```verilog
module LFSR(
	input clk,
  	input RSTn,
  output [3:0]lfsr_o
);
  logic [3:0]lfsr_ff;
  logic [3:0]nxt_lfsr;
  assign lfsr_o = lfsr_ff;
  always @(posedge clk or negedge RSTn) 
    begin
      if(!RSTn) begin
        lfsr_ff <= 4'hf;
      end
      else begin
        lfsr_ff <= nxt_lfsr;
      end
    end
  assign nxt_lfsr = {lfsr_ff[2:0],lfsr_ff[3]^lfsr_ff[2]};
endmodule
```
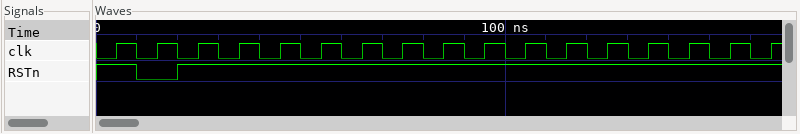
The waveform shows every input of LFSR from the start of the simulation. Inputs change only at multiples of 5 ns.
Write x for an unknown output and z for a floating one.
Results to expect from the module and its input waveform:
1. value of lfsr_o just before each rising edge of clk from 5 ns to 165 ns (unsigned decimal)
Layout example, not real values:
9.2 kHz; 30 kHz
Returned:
x, 15, 15, 14, 12, 8, 1, 2, 4, 9, 3, 6, 13, 10, 5, 11, 7
